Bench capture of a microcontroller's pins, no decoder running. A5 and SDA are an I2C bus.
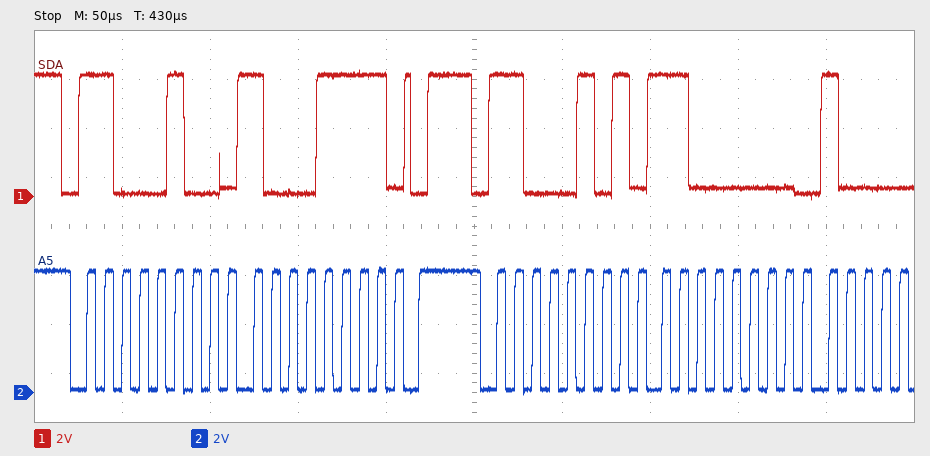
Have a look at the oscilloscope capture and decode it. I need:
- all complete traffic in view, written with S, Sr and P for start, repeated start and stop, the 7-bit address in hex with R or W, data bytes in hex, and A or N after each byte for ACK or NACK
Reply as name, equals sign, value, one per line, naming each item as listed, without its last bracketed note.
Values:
all complete traffic in view, written with S, Sr and P for start, repeated start and stop, the 7-bit address in hex with R or W, data bytes in hex, and A or N after each byte for ACK or NACK = S 62W A 8F A P S 62R A C0 A
